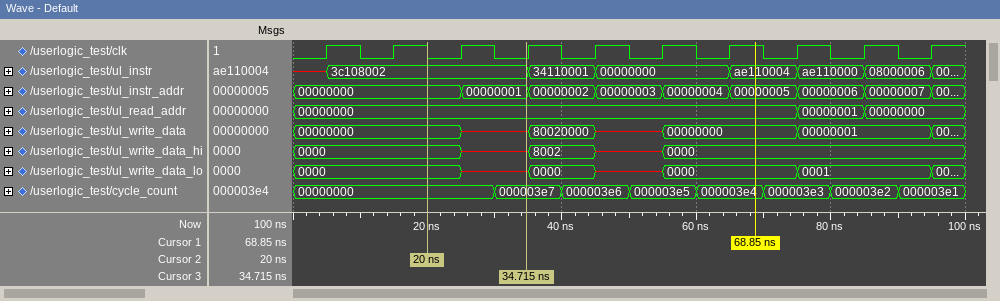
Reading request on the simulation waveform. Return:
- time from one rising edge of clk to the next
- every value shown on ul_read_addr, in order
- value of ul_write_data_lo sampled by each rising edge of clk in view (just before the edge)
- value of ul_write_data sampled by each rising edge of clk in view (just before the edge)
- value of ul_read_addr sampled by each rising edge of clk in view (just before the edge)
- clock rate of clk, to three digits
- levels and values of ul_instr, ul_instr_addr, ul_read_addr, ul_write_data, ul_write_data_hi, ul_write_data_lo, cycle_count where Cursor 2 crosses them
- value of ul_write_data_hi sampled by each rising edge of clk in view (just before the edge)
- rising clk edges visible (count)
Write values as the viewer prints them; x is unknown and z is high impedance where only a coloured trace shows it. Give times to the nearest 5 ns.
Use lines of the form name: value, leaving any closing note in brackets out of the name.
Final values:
time from one rising edge of clk to the next: 10 ns
every value shown on ul_read_addr, in order: 00000000, 00000001, 00000000
value of ul_write_data_lo sampled by each rising edge of clk in view: 0000, 0000, 0000, x, 0000, x, 0000, 0000, 0001, 0001
value of ul_write_data sampled by each rising edge of clk in view: 00000000, 00000000, 00000000, x, 80020000, x, 00000000, 00000000, 00000001, 00000001
value of ul_read_addr sampled by each rising edge of clk in view: 00000000, 00000000, 00000000, 00000000, 00000000, 00000000, 00000000, 00000000, 00000001, 00000000
clock rate of clk, to three digits: 100 MHz
levels and values of ul_instr, ul_instr_addr, ul_read_addr, ul_write_data, ul_write_data_hi, ul_write_data_lo, cycle_count where Cursor 2 crosses them: ul_instr=3c108002, ul_instr_addr=00000000, ul_read_addr=00000000, ul_write_data=00000000, ul_write_data_hi=0000, ul_write_data_lo=0000, cycle_count=00000000
value of ul_write_data_hi sampled by each rising edge of clk in view: 0000, 0000, 0000, x, 8002, x, 0000, 0000, 0000, 0000
rising clk edges visible: 10
